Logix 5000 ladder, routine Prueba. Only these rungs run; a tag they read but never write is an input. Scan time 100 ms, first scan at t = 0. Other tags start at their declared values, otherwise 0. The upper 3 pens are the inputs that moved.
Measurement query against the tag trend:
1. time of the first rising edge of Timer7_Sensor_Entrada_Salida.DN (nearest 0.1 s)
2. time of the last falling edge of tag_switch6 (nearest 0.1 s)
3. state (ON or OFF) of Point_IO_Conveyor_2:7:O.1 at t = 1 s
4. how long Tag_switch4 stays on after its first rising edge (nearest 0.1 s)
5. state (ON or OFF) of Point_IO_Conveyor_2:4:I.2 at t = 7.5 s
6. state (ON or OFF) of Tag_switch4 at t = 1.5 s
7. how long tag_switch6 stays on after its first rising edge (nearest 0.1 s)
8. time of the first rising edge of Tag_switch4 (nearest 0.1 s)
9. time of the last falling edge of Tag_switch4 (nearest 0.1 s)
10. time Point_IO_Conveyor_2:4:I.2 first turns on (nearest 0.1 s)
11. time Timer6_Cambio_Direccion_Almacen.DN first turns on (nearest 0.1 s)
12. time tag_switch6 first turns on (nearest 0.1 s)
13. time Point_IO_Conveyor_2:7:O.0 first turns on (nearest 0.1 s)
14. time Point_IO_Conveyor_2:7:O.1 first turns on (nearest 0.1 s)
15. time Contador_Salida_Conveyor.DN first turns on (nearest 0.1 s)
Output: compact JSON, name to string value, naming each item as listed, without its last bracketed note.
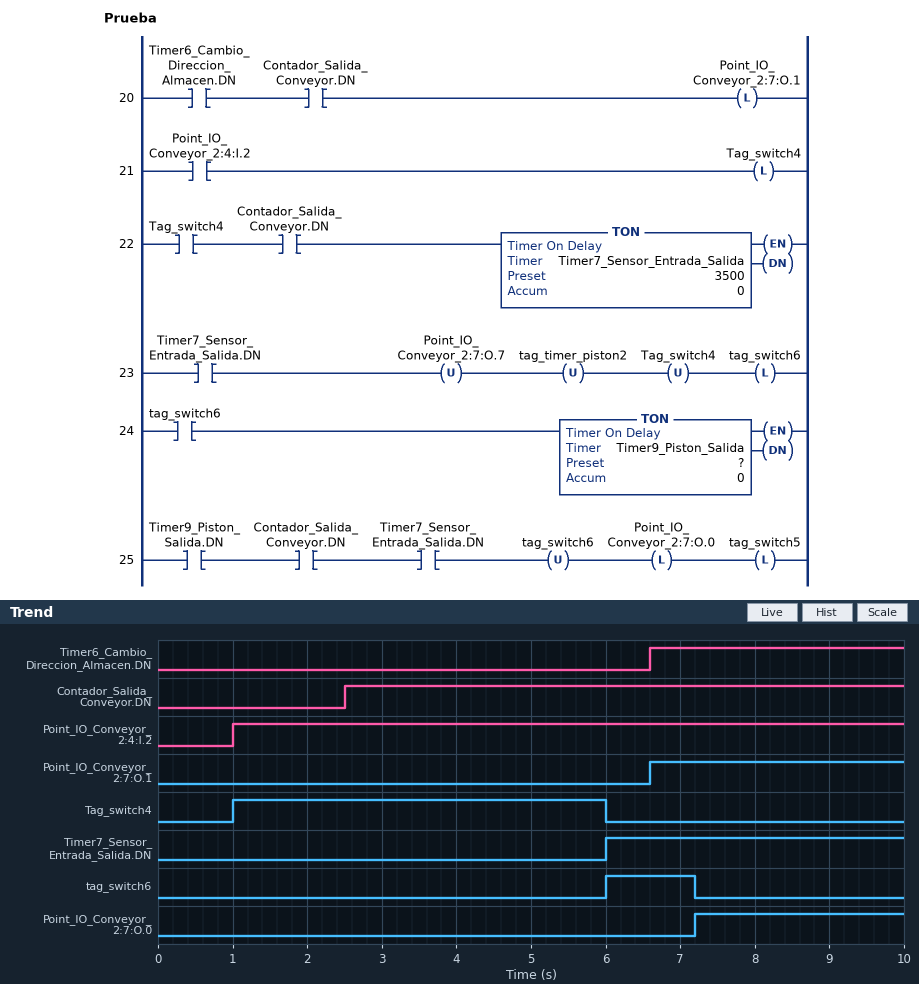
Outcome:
{"time of the first rising edge of Timer7_Sensor_Entrada_Salida.DN": "6.0 s", "time of the last falling edge of tag_switch6": "7.2 s", "state (ON or OFF) of Point_IO_Conveyor_2:7:O.1 at t = 1 s": "OFF", "how long Tag_switch4 stays on after its first rising edge": "5.0 s", "state (ON or OFF) of Point_IO_Conveyor_2:4:I.2 at t = 7.5 s": "ON", "state (ON or OFF) of Tag_switch4 at t = 1.5 s": "ON", "how long tag_switch6 stays on after its first rising edge": "1.2 s", "time of the first rising edge of Tag_switch4": "1.0 s", "time of the last falling edge of Tag_switch4": "6.0 s", "time Point_IO_Conveyor_2:4:I.2 first turns on": "1.0 s", "time Timer6_Cambio_Direccion_Almacen.DN first turns on": "6.6 s", "time tag_switch6 first turns on": "6.0 s", "time Point_IO_Conveyor_2:7:O.0 first turns on": "7.2 s", "time Point_IO_Conveyor_2:7:O.1 first turns on": "6.6 s", "time Contador_Salida_Conveyor.DN first turns on": "2.5 s"}
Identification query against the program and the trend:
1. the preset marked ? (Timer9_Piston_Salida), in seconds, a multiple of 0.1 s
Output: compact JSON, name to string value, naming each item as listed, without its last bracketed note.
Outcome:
{"the preset marked ? (Timer9_Piston_Salida), in seconds, a multiple of 0.1 s": "1.2 s"}
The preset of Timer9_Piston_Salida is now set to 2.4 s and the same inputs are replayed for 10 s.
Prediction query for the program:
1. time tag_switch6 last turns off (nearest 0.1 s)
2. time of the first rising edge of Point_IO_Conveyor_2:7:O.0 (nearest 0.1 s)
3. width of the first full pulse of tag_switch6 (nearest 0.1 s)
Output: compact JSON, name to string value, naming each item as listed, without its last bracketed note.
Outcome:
{"time tag_switch6 last turns off": "8.4 s", "time of the first rising edge of Point_IO_Conveyor_2:7:O.0": "8.4 s", "width of the first full pulse of tag_switch6": "2.4 s"}
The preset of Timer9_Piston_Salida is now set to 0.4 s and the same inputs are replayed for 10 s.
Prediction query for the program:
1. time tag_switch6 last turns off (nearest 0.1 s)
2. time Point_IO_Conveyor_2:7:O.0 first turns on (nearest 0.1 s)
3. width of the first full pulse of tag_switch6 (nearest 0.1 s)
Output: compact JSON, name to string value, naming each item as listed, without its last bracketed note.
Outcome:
{"time tag_switch6 last turns off": "6.4 s", "time Point_IO_Conveyor_2:7:O.0 first turns on": "6.4 s", "width of the first full pulse of tag_switch6": "0.4 s"}
